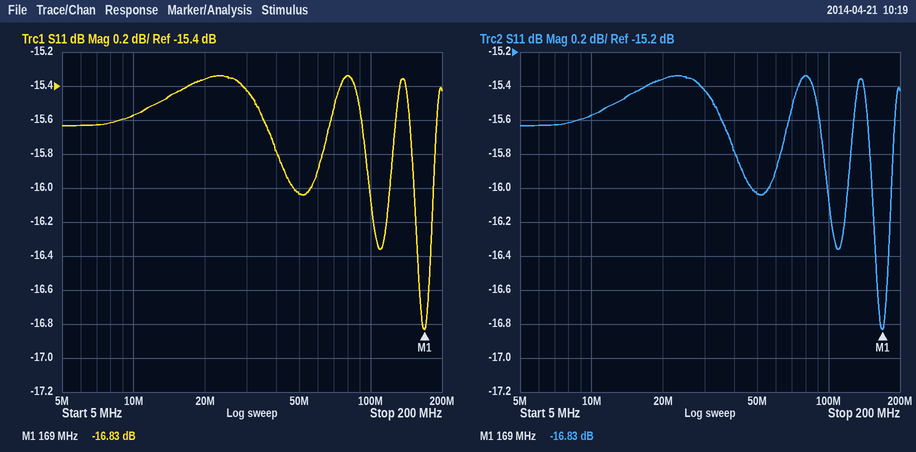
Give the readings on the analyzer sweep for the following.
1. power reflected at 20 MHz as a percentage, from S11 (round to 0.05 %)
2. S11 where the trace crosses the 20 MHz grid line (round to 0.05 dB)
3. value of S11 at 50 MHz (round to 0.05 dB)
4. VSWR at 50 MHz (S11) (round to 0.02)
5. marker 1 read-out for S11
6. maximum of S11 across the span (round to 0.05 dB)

2.90 %
-15.35 dB
-16.05 dB
1.38
-16.83 dB
-15.35 dB
